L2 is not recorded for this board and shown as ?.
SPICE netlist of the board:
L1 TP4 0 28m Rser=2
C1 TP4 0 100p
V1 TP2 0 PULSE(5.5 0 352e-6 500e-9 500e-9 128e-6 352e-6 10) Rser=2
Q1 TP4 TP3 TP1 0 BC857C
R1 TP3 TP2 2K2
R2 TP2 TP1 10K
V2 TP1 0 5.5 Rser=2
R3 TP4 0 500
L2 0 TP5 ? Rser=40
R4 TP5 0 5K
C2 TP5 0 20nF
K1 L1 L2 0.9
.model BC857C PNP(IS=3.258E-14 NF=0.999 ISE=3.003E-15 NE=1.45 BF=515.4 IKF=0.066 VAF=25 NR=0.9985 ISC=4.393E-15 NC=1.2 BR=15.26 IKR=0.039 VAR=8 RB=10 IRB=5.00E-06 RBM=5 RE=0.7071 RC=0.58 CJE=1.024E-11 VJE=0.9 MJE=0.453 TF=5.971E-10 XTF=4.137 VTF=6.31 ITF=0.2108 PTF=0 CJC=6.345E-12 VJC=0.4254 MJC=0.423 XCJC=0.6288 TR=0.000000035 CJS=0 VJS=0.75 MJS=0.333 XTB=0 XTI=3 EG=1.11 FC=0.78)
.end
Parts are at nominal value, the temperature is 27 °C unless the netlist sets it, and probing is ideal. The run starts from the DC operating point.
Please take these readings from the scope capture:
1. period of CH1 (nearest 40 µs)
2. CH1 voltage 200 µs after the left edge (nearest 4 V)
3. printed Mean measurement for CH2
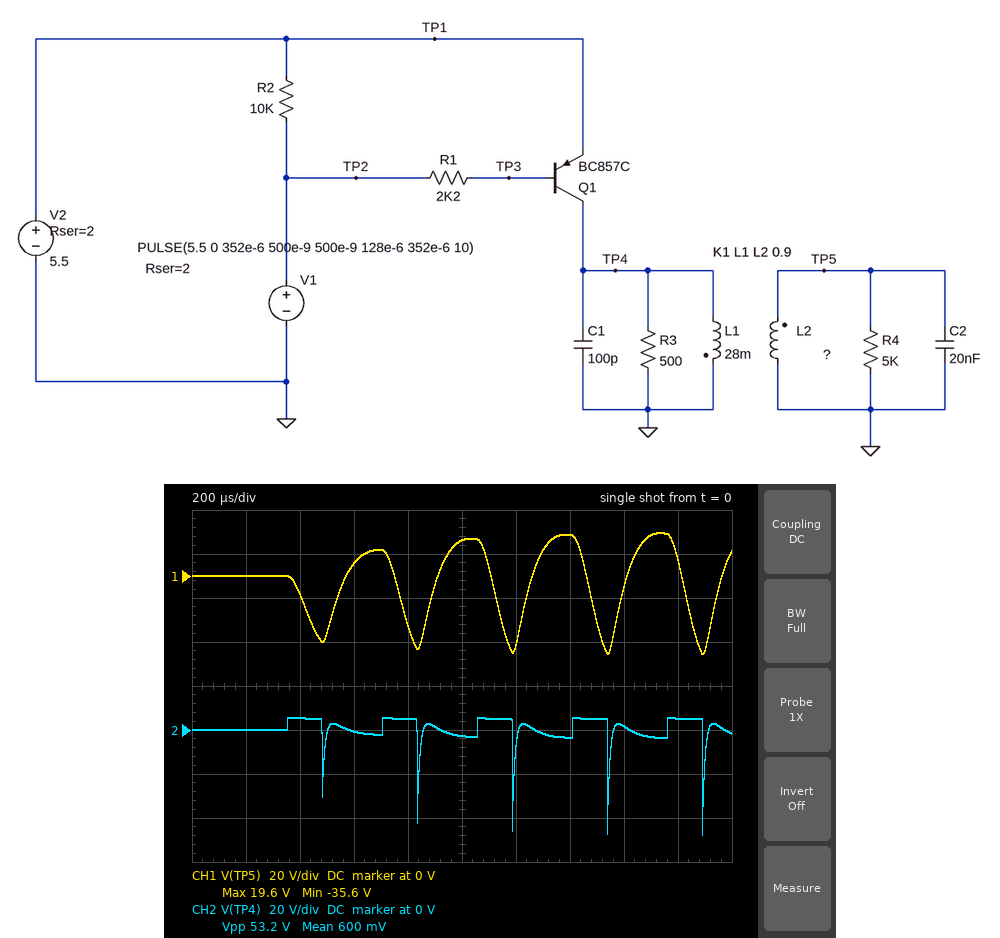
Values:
360 µs
0 V
600 mV
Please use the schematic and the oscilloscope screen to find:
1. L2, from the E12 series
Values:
680 mH
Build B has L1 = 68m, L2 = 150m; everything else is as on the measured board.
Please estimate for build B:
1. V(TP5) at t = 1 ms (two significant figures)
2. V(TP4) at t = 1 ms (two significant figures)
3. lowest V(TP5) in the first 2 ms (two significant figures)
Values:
2.8 V
-2.3 V
-13 V
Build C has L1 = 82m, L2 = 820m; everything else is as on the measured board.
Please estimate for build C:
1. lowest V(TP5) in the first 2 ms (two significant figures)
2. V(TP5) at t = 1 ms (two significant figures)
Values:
-21 V
9.0 V
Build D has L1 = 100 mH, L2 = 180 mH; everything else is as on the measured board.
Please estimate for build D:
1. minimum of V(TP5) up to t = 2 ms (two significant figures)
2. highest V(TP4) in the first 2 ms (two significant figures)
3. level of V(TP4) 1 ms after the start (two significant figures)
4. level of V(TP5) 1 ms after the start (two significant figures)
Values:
-12 V
5.4 V
-2.4 V
2.2 V
